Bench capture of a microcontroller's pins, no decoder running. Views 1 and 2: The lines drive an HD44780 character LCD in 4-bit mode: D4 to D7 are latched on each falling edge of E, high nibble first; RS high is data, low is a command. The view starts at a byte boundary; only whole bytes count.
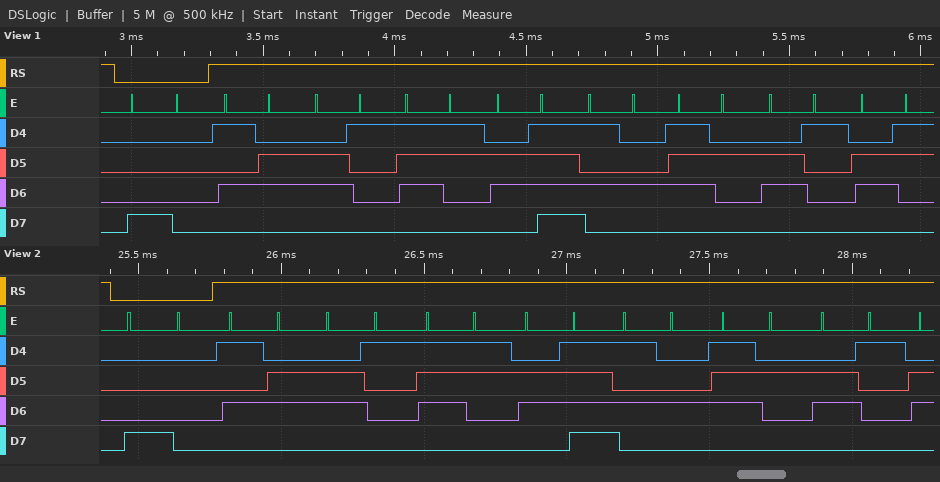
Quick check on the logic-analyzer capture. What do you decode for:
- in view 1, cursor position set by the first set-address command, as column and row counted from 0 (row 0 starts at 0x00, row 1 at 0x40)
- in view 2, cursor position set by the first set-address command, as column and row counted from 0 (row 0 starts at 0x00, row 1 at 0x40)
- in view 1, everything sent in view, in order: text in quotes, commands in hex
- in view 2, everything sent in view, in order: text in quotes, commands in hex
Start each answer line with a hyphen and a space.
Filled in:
- column 0, row 0
- column 0, row 0
- 0x80 "VasoTrac"
- 0x80 "VasoTra"
